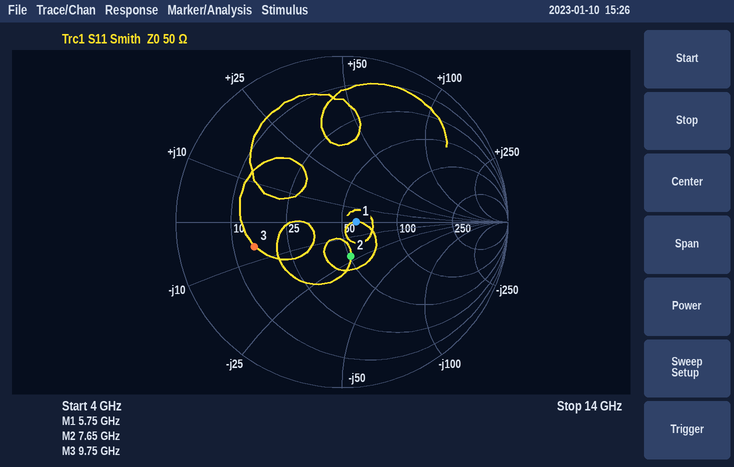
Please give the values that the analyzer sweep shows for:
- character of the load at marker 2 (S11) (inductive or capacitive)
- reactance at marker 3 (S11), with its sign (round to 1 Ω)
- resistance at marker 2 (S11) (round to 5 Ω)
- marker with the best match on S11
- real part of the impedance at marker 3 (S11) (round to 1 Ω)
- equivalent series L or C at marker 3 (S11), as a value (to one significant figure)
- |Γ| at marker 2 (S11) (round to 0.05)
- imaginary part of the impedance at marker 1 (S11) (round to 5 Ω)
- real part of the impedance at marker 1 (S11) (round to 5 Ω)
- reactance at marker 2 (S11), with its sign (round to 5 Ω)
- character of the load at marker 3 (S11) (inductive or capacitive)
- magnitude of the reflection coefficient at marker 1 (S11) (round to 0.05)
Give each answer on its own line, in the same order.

capacitive
-6 Ω
50 Ω
marker 1
15 Ω
3 pF
0.20
0 Ω
60 Ω
-20 Ω
capacitive
0.10
